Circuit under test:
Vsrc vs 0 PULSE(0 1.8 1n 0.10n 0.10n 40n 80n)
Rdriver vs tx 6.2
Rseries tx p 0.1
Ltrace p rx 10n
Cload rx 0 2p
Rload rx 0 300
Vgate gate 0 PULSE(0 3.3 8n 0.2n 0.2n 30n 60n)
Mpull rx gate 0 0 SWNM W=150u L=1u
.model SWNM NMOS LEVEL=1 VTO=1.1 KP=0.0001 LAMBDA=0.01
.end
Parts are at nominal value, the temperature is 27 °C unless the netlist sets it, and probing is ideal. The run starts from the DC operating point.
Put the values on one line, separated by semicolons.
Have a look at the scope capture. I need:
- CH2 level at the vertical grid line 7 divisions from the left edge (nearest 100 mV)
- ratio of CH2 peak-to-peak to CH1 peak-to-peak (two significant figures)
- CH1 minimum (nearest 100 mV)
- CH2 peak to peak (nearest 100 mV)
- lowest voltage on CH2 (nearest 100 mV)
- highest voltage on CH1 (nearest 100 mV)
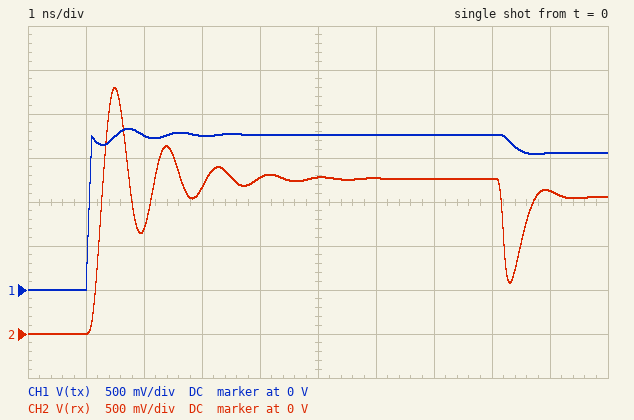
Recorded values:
1.8 V; 1.5; 0 V; 2.8 V; 0 V; 1.8 V
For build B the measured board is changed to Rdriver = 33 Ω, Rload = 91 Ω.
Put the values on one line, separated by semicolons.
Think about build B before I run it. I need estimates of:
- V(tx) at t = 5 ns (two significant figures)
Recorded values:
1.3 V
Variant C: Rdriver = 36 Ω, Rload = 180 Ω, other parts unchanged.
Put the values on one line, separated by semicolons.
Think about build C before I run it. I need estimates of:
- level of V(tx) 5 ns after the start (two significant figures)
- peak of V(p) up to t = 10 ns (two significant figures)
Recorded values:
1.5 V; 1.6 V
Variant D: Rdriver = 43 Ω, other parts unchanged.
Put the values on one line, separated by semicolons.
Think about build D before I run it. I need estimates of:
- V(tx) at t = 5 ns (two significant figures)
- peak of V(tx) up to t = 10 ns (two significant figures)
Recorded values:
1.6 V; 1.7 V
